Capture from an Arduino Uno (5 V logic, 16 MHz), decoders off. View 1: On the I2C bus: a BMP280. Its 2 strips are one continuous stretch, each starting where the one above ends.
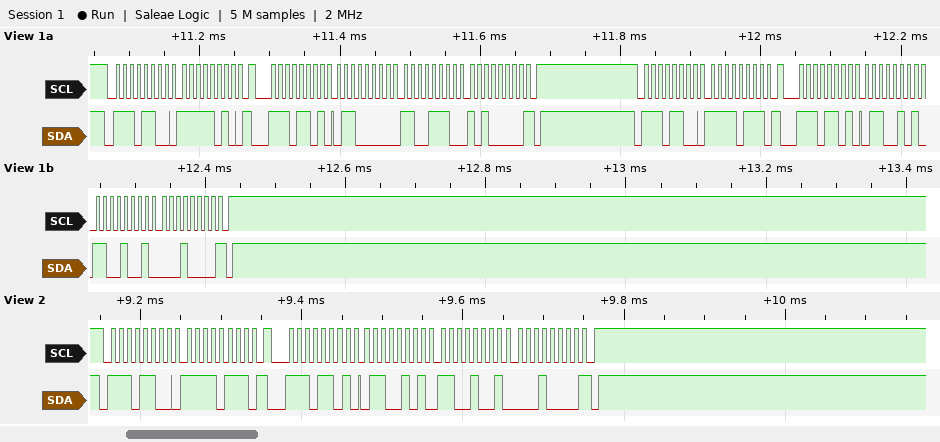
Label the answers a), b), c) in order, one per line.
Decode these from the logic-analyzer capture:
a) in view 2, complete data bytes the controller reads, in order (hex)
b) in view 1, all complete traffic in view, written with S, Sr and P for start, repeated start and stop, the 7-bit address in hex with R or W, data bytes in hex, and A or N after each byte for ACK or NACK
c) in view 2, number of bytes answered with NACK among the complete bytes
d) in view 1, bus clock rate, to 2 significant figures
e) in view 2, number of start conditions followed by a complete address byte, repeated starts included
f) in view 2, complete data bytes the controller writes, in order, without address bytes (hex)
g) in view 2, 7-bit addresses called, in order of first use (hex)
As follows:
a) 65 C9 10
b) S 76W A FA A Sr 76R A 60 A CE A A0 N P S 76W A F7 A Sr 76R A 65 A C9 A 10 N P
c) 1
d) 100 kHz
e) 2
f) F7
g) 0x76
